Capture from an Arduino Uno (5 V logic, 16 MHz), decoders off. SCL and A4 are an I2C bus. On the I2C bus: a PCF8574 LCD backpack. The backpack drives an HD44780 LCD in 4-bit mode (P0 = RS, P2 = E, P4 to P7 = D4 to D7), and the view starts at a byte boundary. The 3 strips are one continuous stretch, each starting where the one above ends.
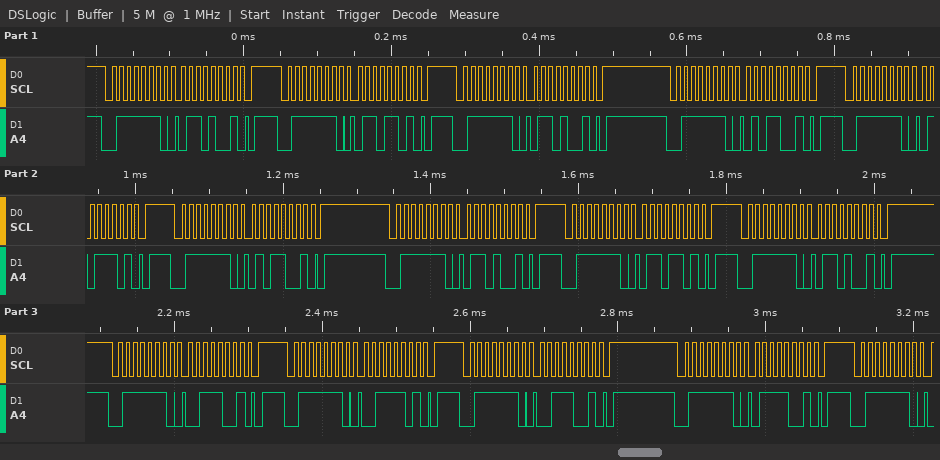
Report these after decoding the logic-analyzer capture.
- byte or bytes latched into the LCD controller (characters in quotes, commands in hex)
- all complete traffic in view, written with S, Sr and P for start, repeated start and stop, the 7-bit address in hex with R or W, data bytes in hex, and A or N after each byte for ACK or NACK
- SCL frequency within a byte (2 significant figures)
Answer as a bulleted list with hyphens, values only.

- 'e' 'c'
- S 3FW A 69 A P S 3FW A 6D A P S 3FW A 69 A P S 3FW A 59 A P S 3FW A 5D A P S 3FW A 59 A P S 3FW A 69 A P S 3FW A 6D A P S 3FW A 69 A P S 3FW A 39 A P S 3FW A 3D A P S 3FW A 39 A P S 3FW A 79 A P S 3FW A
- 100 kHz
